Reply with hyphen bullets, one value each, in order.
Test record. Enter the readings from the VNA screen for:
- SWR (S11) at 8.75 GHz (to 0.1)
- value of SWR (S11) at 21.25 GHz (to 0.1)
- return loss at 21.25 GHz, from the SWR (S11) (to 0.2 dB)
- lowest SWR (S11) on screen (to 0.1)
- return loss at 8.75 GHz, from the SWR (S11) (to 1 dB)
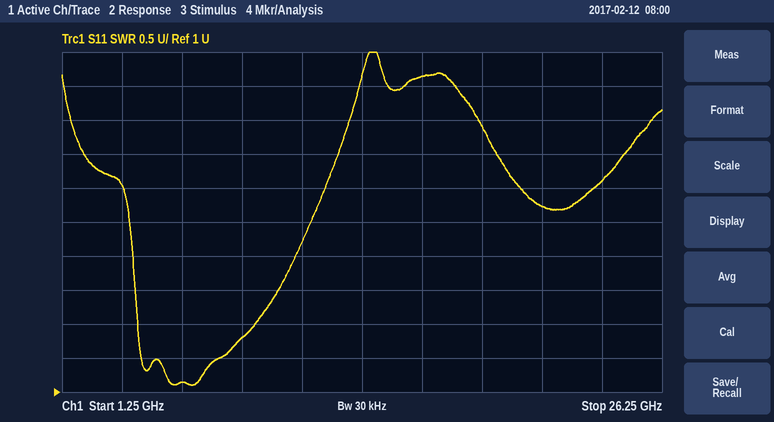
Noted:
- 1.8
- 3.7
- 4.8 dB
- 1.1
- 11 dB
